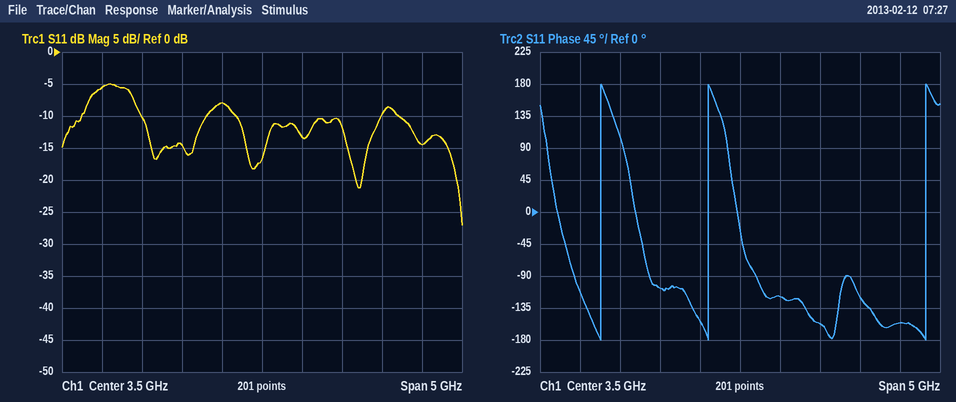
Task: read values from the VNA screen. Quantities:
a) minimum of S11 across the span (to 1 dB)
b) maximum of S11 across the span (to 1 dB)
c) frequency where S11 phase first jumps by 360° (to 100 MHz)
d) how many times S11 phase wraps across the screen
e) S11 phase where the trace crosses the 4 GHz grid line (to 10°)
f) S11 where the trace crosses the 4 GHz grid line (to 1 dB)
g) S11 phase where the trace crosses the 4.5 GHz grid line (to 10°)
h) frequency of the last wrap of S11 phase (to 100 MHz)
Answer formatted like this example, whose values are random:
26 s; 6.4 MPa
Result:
-27 dB; -5 dB; 1.8 GHz; 3; -120°; -13 dB; -160°; 5.8 GHz
